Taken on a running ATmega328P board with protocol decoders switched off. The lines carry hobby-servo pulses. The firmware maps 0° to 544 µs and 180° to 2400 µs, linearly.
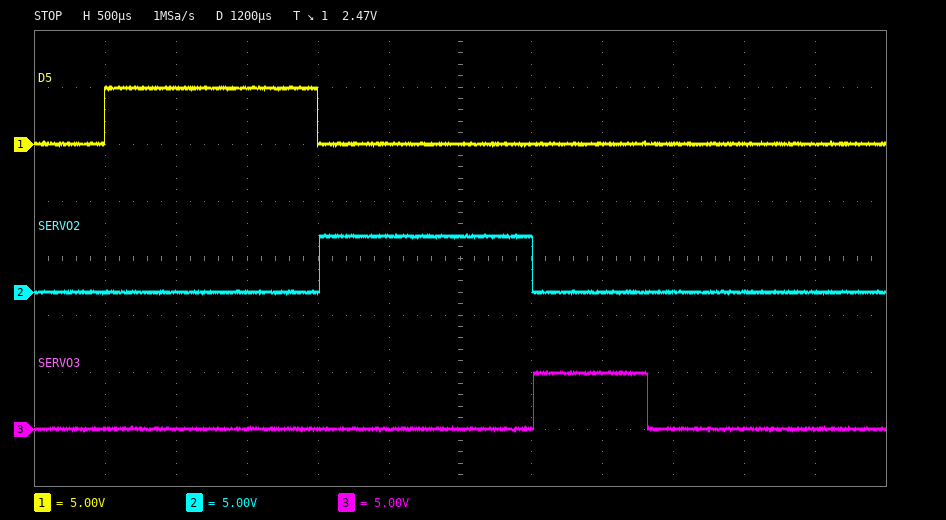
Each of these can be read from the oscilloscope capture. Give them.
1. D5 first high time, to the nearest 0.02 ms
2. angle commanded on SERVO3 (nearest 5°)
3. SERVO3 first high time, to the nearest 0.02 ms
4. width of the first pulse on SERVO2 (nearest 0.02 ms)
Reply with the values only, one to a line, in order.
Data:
1.50 ms
25°
0.80 ms
1.50 ms
